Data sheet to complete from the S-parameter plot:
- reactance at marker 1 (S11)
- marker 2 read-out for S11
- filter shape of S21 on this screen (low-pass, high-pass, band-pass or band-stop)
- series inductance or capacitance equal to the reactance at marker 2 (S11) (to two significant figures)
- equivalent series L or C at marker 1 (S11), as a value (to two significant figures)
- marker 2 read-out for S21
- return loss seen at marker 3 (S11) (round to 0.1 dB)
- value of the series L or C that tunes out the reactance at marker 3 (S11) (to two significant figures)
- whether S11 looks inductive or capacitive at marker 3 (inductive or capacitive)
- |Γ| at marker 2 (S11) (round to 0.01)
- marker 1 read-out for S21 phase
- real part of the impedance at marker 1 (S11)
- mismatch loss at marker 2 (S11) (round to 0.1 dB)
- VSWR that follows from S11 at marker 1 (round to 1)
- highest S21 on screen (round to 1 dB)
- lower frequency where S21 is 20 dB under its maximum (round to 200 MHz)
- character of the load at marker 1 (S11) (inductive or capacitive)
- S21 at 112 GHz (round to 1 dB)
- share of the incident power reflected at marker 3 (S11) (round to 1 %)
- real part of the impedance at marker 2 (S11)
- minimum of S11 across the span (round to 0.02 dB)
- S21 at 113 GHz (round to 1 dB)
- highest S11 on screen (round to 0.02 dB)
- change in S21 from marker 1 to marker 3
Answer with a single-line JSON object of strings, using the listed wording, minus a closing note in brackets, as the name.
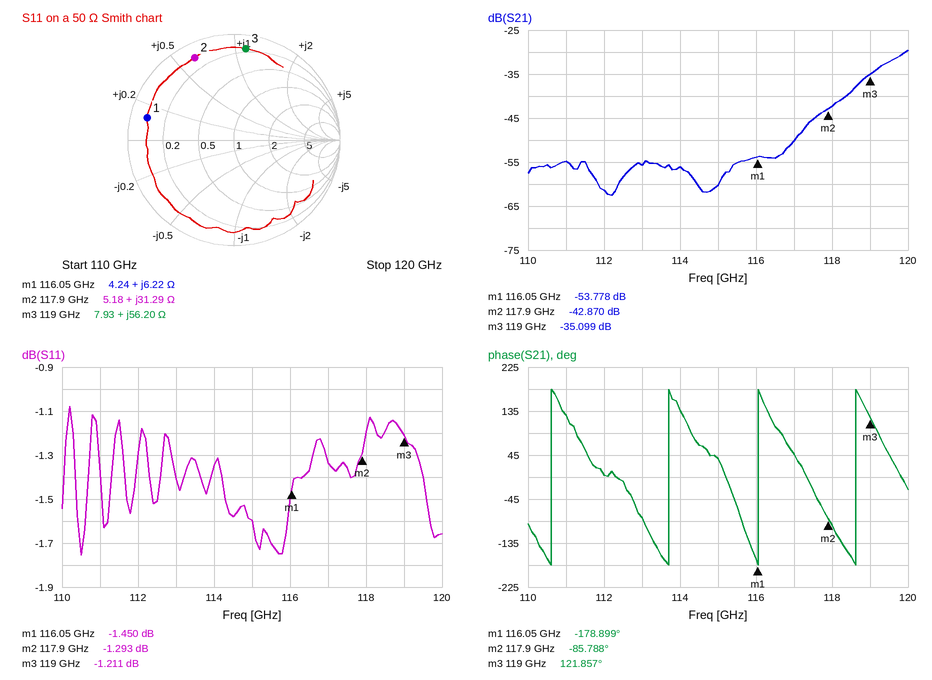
{"reactance at marker 1": "+6.22 Ω", "marker 2 read-out for S11": "-1.293 dB", "filter shape of S21 on this screen": "high-pass", "series inductance or capacitance equal to the reactance at marker 2 (S11)": "42 pH", "equivalent series L or C at marker 1 (S11), as a value": "8.5 pH", "marker 2 read-out for S21": "-42.870 dB", "return loss seen at marker 3 (S11)": "1.2 dB", "value of the series L or C that tunes out the reactance at marker 3 (S11)": "24 fF", "whether S11 looks inductive or capacitive at marker 3": "inductive", "|Γ| at marker 2 (S11)": "0.86", "marker 1 read-out for S21 phase": "-178.899°", "real part of the impedance at marker 1": "4.24 Ω", "mismatch loss at marker 2 (S11)": "5.9 dB", "VSWR that follows from S11 at marker 1": "12", "highest S21 on screen": "-30 dB", "lower frequency where S21 is 20 dB under its maximum": "117.0 GHz", "character of the load at marker 1 (S11)": "inductive", "S21 at 112 GHz": "-61 dB", "share of the incident power reflected at marker 3 (S11)": "76 %", "real part of the impedance at marker 2": "5.18 Ω", "minimum of S11 across the span": "-1.76 dB", "S21 at 113 GHz": "-56 dB", "highest S11 on screen": "-1.08 dB", "change in S21 from marker 1 to marker 3": "18.679 dB"}
